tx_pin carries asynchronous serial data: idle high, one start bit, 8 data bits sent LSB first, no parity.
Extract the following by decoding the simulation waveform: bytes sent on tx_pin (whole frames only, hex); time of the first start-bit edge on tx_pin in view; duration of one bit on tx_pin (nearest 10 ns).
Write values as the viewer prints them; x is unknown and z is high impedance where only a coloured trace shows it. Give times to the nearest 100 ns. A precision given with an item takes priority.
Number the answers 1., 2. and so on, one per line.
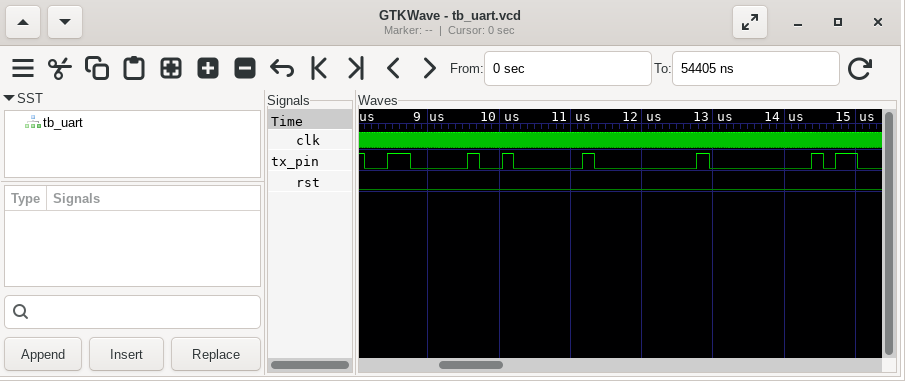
1. 06, 02, 00, 00
2. 8100 ns
3. 160 ns
